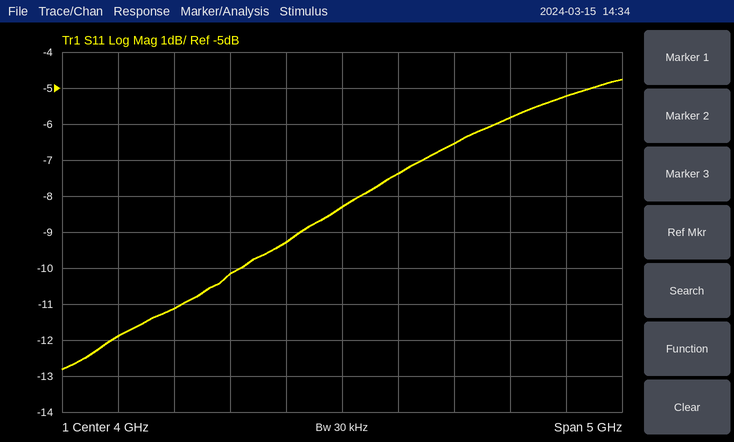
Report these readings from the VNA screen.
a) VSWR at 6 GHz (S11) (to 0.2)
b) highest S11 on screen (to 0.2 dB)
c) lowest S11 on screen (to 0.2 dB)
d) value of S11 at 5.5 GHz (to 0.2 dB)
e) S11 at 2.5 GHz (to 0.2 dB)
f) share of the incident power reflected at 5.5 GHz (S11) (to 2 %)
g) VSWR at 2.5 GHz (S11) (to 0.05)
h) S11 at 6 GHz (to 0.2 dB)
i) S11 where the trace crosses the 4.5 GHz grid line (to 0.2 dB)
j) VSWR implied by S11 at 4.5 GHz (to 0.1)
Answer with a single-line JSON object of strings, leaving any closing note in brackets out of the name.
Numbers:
{"VSWR at 6 GHz (S11)": "3.4", "highest S11 on screen": "-4.8 dB", "lowest S11 on screen": "-12.8 dB", "value of S11 at 5.5 GHz": "-5.8 dB", "S11 at 2.5 GHz": "-11.2 dB", "share of the incident power reflected at 5.5 GHz (S11)": "26 %", "VSWR at 2.5 GHz (S11)": "1.75", "S11 at 6 GHz": "-5.2 dB", "S11 where the trace crosses the 4.5 GHz grid line": "-7.4 dB", "VSWR implied by S11 at 4.5 GHz": "2.5"}
